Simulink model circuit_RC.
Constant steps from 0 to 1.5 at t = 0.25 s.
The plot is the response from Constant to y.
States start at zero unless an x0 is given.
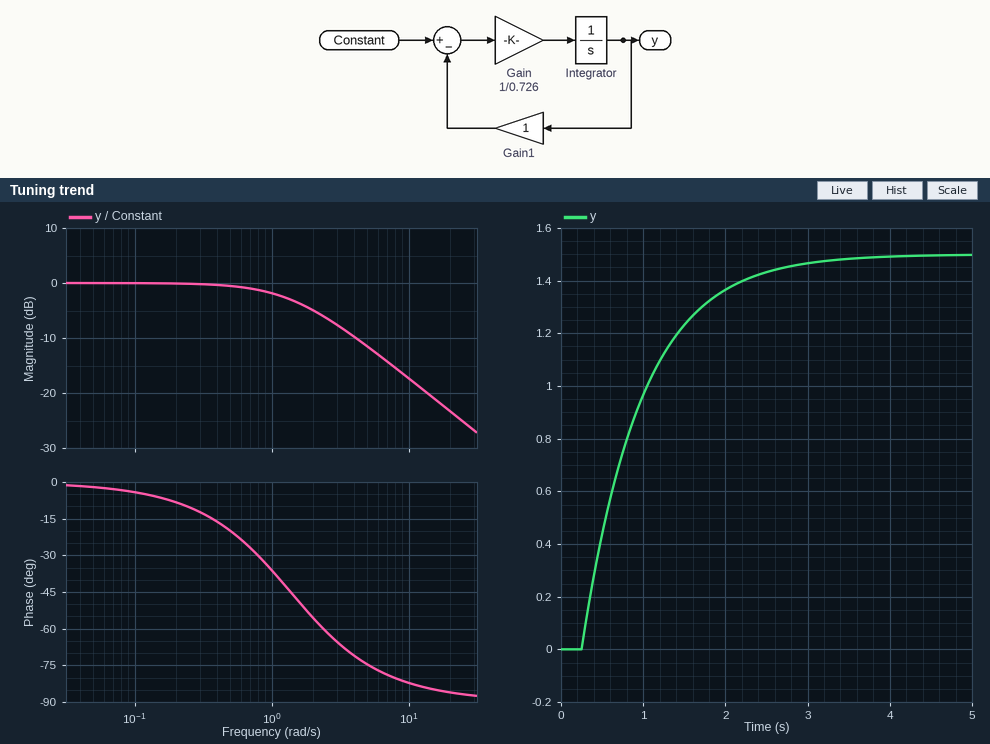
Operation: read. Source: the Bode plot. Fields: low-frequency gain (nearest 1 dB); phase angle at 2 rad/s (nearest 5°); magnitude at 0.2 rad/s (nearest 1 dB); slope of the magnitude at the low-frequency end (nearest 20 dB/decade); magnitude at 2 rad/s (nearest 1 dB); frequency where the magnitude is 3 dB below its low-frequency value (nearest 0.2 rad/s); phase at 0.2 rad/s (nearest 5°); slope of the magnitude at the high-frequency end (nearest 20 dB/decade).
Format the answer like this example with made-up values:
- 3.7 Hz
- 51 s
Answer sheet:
- 0 dB
- -55°
- 0 dB
- 0 dB/decade
- -5 dB
- 1.4 rad/s
- -10°
- -20 dB/decade
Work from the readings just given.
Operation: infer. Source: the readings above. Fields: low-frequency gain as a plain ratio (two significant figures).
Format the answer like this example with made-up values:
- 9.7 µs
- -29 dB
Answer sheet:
- 1.0
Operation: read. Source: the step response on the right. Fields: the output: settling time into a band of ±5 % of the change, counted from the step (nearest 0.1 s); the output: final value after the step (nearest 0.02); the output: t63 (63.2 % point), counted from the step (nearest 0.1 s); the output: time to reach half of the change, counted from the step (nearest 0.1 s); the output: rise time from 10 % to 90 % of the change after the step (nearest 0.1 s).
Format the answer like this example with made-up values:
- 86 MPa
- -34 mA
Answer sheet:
- 2.2 s
- 1.50
- 0.7 s
- 0.5 s
- 1.6 s
